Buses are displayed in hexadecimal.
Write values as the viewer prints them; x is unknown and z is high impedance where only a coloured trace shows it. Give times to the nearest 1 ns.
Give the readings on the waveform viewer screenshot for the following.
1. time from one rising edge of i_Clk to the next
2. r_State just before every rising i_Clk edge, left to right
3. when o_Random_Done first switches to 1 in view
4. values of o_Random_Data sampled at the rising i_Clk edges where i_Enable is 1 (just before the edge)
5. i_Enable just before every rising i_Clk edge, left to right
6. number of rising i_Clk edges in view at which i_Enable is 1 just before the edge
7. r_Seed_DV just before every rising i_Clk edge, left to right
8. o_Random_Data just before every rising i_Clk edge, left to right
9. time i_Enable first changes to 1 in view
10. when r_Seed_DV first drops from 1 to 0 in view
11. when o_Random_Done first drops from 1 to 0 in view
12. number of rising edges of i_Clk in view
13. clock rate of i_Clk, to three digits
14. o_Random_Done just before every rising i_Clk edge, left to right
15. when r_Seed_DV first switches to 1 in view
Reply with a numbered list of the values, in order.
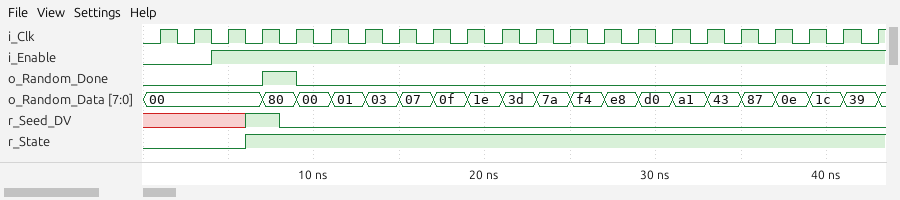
1. 2 ns
2. 0 0 0 1 1 1 1 1 1 1 1 1 1 1 1 1 1 1 1 1 1 1
3. 7 ns
4. 00, 00, 80, 00, 01, 03, 07, 0f, 1e, 3d, 7a, f4, e8, d0, a1, 43, 87, 0e, 1c, 39
5. 0 0 1 1 1 1 1 1 1 1 1 1 1 1 1 1 1 1 1 1 1 1
6. 20
7. x x x 1 0 0 0 0 0 0 0 0 0 0 0 0 0 0 0 0 0 0
8. 00, 00, 00, 00, 80, 00, 01, 03, 07, 0f, 1e, 3d, 7a, f4, e8, d0, a1, 43, 87, 0e, 1c, 39
9. 4 ns
10. 8 ns
11. 9 ns
12. 22
13. 500 MHz
14. 0 0 0 0 1 0 0 0 0 0 0 0 0 0 0 0 0 0 0 0 0 0
15. 6 ns
